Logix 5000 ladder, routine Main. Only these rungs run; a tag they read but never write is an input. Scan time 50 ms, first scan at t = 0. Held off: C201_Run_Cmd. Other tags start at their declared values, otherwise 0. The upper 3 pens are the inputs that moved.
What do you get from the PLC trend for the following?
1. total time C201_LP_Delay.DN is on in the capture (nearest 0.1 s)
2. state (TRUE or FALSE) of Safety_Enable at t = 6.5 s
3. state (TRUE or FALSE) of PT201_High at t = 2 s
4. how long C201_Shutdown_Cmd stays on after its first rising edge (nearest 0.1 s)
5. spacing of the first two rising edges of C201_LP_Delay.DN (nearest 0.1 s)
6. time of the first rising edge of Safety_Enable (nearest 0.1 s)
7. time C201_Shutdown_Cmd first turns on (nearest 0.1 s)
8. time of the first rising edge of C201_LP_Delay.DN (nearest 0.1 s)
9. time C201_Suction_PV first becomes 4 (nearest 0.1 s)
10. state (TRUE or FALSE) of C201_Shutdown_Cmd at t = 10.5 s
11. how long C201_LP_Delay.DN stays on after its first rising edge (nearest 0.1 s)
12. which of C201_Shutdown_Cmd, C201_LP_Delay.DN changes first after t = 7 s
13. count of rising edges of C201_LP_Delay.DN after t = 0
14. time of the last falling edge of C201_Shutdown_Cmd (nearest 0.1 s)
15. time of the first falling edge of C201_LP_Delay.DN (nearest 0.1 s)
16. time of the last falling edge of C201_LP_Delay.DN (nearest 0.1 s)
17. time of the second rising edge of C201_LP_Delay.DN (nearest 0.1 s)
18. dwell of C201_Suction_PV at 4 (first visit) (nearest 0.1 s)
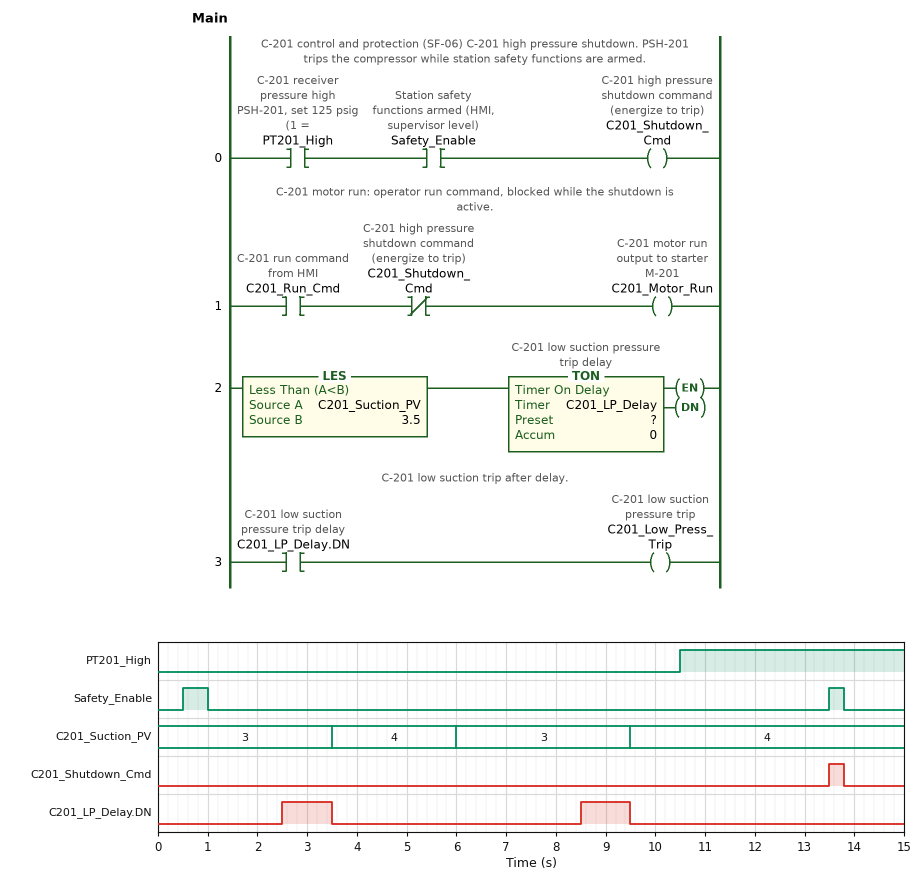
2.0 s
FALSE
FALSE
0.3 s
6.0 s
0.5 s
13.5 s
2.5 s
3.5 s
FALSE
1.0 s
C201_LP_Delay.DN
2
13.8 s
3.5 s
9.5 s
8.5 s
2.5 s
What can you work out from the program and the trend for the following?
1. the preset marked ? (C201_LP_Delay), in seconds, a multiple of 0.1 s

2.5 s
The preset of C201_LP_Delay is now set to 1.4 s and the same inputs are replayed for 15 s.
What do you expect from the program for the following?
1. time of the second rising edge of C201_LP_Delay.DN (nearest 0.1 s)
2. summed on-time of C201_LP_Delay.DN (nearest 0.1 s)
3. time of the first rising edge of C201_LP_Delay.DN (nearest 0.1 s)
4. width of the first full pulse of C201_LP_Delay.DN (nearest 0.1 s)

7.4 s
4.2 s
1.4 s
2.1 s
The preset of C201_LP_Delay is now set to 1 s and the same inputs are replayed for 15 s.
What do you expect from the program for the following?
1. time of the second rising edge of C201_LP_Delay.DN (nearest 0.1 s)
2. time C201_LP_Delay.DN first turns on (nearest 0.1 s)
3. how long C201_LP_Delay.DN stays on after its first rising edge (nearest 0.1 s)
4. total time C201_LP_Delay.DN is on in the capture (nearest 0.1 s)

7.0 s
1.0 s
2.5 s
5.0 s
